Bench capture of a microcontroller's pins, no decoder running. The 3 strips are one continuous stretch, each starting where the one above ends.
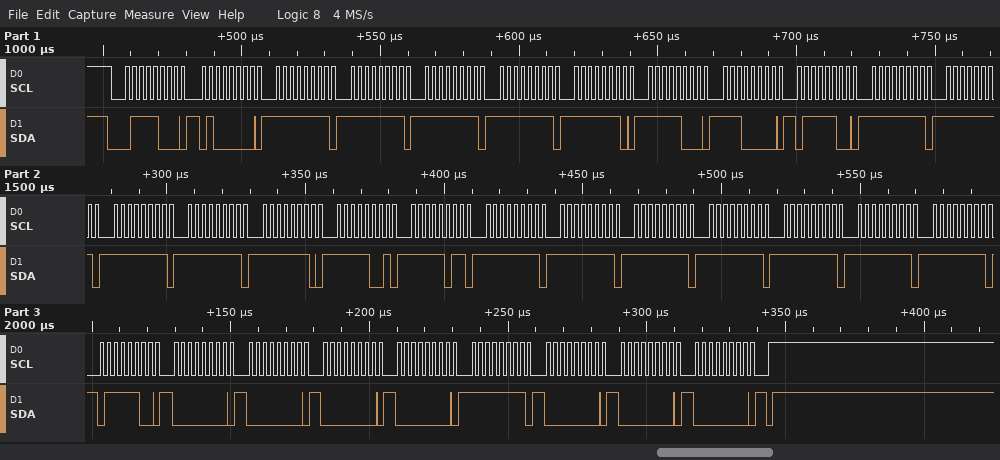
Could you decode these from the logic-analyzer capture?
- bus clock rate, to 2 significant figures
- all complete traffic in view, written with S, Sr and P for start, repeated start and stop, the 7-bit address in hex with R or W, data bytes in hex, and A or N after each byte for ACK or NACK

400 kHz
S 3CW A 40 A FF A FF A FF A FF A FE A F8 A E0 A 7C A FF A FF A FF A FF A FE A F9 A FB A FF A FF A FF A FF A FF A FF A FF A 7C A 00 A 00 A 00 A 00 A FF A 00 A 00 A 00 A P
